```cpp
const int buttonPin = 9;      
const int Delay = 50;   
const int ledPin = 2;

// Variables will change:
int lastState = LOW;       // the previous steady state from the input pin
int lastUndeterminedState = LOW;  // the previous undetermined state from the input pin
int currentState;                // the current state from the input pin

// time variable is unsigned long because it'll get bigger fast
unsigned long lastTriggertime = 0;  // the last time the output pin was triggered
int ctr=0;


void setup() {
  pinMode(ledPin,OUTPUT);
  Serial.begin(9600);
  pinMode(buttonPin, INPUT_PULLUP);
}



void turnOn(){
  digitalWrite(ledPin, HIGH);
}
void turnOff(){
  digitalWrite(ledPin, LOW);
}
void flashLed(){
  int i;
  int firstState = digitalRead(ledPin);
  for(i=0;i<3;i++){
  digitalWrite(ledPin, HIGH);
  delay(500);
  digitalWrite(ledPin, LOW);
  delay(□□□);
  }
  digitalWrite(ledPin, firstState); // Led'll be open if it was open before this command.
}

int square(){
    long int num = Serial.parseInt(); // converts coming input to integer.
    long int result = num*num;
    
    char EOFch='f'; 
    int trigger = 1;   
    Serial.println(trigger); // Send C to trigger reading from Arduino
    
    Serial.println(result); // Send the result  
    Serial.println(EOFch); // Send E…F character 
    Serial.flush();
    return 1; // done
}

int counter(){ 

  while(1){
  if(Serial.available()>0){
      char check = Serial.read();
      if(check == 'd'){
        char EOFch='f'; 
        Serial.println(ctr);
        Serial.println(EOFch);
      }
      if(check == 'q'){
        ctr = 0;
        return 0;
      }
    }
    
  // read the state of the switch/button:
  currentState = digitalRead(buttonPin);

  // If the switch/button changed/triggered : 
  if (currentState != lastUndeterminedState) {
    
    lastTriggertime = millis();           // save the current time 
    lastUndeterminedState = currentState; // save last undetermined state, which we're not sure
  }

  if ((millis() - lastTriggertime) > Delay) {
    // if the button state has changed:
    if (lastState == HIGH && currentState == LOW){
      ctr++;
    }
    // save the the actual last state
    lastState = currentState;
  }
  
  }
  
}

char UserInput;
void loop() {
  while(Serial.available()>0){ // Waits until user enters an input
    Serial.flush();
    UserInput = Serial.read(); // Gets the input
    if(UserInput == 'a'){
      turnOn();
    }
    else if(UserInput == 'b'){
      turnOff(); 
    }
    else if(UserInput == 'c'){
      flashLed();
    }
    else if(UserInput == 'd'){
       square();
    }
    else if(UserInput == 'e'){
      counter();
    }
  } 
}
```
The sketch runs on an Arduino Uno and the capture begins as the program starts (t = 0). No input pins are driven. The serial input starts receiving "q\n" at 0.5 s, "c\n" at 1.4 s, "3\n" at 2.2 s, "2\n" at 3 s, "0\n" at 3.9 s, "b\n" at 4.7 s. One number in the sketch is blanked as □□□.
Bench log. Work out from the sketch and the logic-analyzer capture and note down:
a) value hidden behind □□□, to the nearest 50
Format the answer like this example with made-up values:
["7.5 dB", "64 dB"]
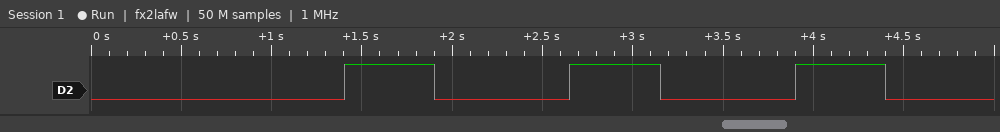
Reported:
["750"]
